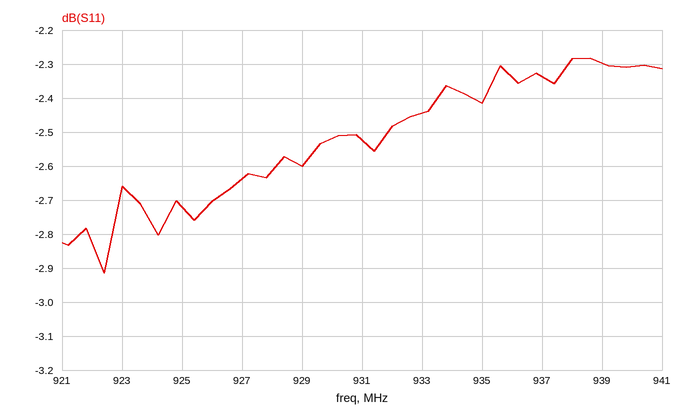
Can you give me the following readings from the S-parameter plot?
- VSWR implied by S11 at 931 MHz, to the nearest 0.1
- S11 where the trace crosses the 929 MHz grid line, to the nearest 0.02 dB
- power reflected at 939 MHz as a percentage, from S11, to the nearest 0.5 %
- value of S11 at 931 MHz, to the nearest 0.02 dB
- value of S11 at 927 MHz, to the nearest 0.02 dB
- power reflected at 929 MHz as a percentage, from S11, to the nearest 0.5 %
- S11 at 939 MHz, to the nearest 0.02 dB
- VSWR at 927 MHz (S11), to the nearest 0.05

6.9
-2.60 dB
59.0 %
-2.52 dB
-2.64 dB
55.0 %
-2.30 dB
6.65
